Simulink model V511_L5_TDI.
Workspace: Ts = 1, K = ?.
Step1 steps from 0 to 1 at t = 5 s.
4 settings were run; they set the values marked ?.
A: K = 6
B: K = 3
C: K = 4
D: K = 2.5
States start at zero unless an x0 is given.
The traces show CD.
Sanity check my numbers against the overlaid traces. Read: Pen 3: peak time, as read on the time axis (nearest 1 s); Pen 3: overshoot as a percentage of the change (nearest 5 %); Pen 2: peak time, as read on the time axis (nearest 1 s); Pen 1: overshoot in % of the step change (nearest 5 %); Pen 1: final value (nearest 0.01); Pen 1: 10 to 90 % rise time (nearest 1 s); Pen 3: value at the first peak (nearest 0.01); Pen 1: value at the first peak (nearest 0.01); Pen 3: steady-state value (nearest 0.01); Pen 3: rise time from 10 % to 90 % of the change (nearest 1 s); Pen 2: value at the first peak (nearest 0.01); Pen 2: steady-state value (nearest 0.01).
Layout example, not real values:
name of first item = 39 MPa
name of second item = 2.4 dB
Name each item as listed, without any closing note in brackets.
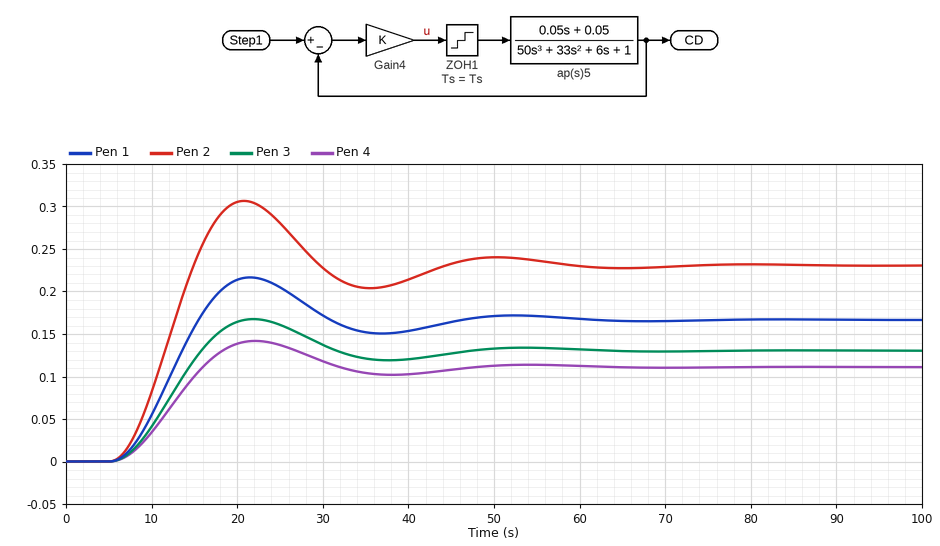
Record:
Pen 3: peak time, as read on the time axis = 22 s
Pen 3: overshoot as a percentage of the change = 30 %
Pen 2: peak time, as read on the time axis = 21 s
Pen 1: overshoot in % of the step change = 30 %
Pen 1: final value = 0.17
Pen 1: 10 to 90 % rise time = 7 s
Pen 3: value at the first peak = 0.17
Pen 1: value at the first peak = 0.22
Pen 3: steady-state value = 0.13
Pen 3: rise time from 10 % to 90 % of the change = 7 s
Pen 2: value at the first peak = 0.31
Pen 2: steady-state value = 0.23
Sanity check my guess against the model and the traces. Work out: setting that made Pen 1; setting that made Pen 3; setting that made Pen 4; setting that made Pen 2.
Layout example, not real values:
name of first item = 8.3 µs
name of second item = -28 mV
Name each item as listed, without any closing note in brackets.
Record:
setting that made Pen 1 = C
setting that made Pen 3 = B
setting that made Pen 4 = D
setting that made Pen 2 = A
